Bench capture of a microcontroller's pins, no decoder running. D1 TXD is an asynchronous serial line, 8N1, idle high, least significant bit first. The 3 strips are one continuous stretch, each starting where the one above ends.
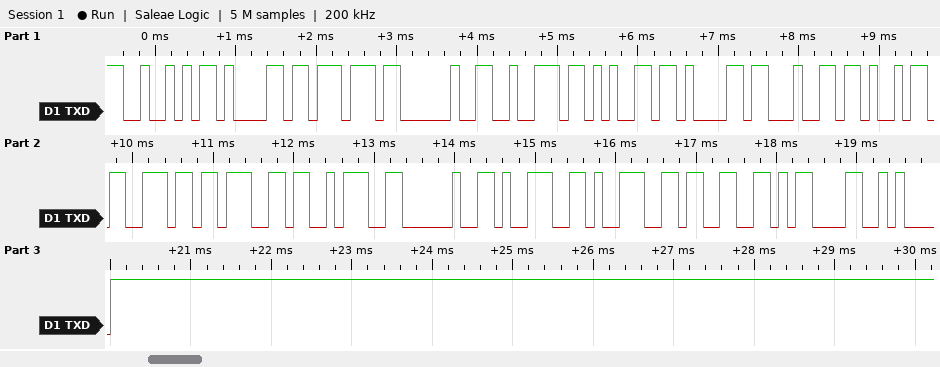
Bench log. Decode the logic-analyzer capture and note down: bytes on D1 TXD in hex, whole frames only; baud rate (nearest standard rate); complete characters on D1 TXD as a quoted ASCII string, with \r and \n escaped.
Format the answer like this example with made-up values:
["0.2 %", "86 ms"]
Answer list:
["52 61 77 20 72 65 61 64 69 6E 67 3A 20 39 39 33 0D 0A", "9600 baud", "\"Raw reading: 993\\r\\n\""]
